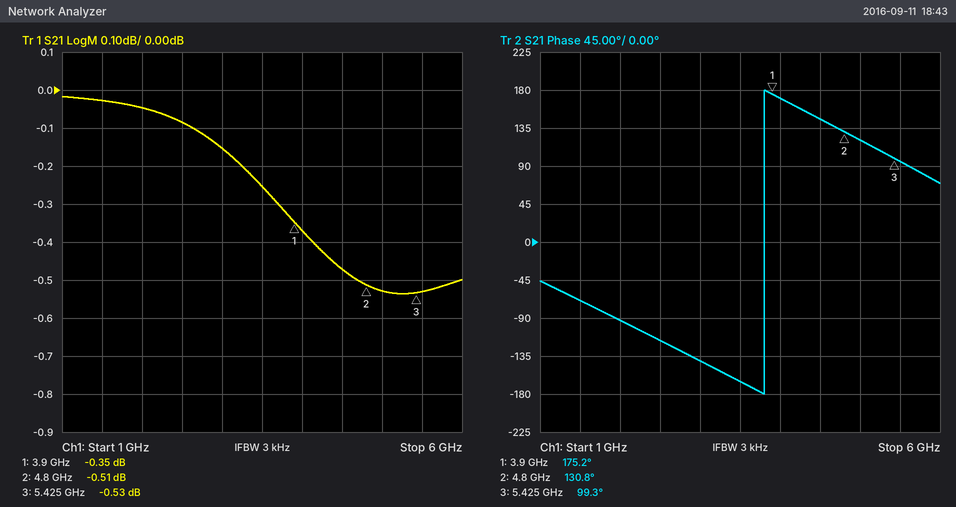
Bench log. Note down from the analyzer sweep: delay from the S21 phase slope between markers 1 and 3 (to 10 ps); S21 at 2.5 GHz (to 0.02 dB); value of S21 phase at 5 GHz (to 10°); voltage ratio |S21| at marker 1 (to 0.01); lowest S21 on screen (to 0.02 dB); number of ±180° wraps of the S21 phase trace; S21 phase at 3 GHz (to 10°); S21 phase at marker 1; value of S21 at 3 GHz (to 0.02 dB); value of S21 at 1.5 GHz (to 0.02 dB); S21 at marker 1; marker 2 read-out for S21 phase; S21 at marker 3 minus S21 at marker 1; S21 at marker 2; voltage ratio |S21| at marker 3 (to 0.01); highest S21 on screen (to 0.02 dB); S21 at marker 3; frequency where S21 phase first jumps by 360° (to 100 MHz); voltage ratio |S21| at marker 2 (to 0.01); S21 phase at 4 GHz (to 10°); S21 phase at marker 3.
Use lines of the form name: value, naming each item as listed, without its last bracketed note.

delay from the S21 phase slope between markers 1 and 3: 140 ps
S21 at 2.5 GHz: -0.08 dB
value of S21 phase at 5 GHz: 120°
voltage ratio |S21| at marker 1: 0.96
lowest S21 on screen: -0.54 dB
number of ±180° wraps of the S21 phase trace: 1
S21 phase at 3 GHz: -140°
S21 phase at marker 1: 175.2°
value of S21 at 3 GHz: -0.16 dB
value of S21 at 1.5 GHz: -0.02 dB
S21 at marker 1: -0.35 dB
marker 2 read-out for S21 phase: 130.8°
S21 at marker 3 minus S21 at marker 1: -0.18 dB
S21 at marker 2: -0.51 dB
voltage ratio |S21| at marker 3: 0.94
highest S21 on screen: -0.02 dB
S21 at marker 3: -0.53 dB
frequency where S21 phase first jumps by 360°: 3.8 GHz
voltage ratio |S21| at marker 2: 0.94
S21 phase at 4 GHz: 170°
S21 phase at marker 3: 99.3°
